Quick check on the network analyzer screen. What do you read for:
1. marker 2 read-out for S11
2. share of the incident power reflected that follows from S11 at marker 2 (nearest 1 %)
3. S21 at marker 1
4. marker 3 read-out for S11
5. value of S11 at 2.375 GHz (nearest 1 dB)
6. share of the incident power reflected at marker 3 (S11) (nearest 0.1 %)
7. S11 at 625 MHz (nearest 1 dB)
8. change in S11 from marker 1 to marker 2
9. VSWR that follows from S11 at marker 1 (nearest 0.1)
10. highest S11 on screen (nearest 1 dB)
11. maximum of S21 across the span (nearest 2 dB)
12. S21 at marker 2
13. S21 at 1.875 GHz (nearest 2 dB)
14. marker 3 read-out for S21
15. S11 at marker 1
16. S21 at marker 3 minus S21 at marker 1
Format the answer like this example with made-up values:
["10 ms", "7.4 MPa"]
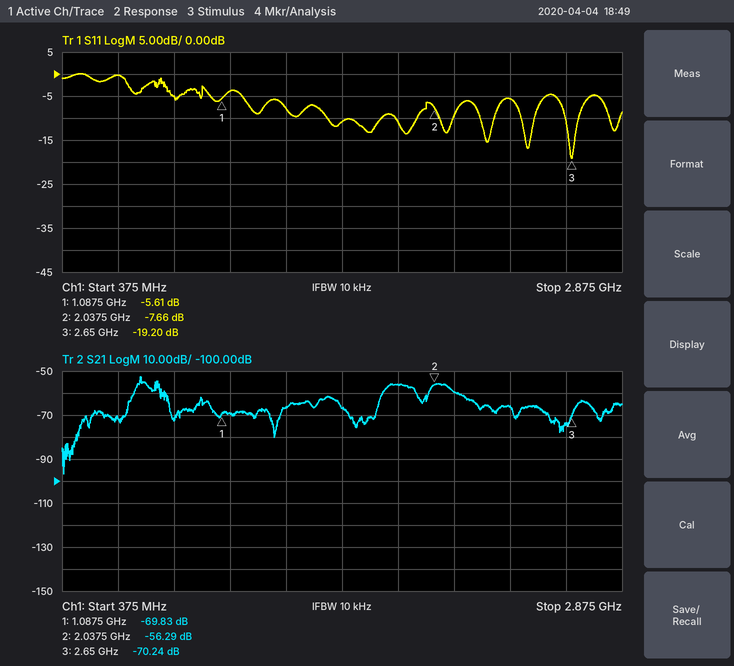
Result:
["-7.66 dB", "17 %", "-69.83 dB", "-19.20 dB", "-6 dB", "1.2 %", "0 dB", "-2.05 dB", "3.2", "0 dB", "-52 dB", "-56.29 dB", "-56 dB", "-70.24 dB", "-5.61 dB", "-0.41 dB"]
